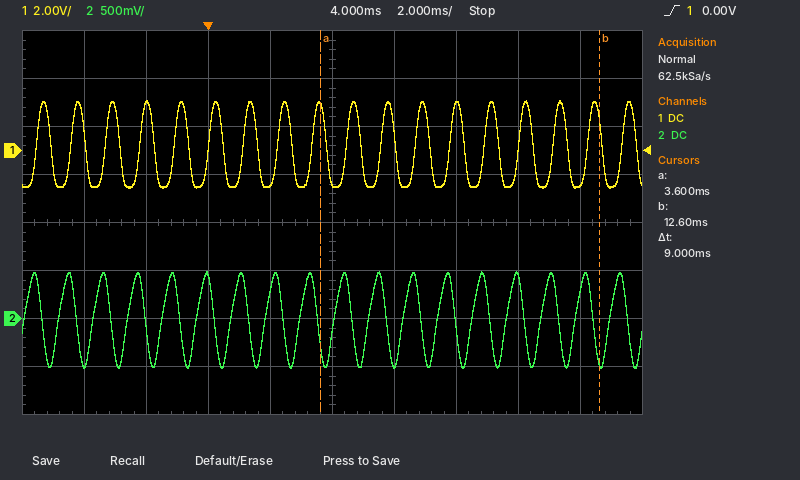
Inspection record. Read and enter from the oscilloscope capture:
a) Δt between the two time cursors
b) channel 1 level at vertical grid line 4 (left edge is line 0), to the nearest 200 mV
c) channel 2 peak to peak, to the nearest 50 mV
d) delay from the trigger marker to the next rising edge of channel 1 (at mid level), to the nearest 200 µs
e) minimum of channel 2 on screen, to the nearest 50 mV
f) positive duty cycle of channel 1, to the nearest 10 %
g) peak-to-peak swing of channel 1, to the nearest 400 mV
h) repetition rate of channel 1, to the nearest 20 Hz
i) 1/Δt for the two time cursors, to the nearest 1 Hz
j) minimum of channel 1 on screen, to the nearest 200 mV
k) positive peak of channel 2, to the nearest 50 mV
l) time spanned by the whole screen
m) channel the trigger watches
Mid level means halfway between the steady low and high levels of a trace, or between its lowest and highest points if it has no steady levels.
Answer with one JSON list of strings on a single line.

["9 ms", "-1.4 V", "1.00 V", "1.2 ms", "-500 mV", "40 %", "3.6 V", "900 Hz", "111 Hz", "-1.6 V", "500 mV", "20 ms", "channel 1"]
